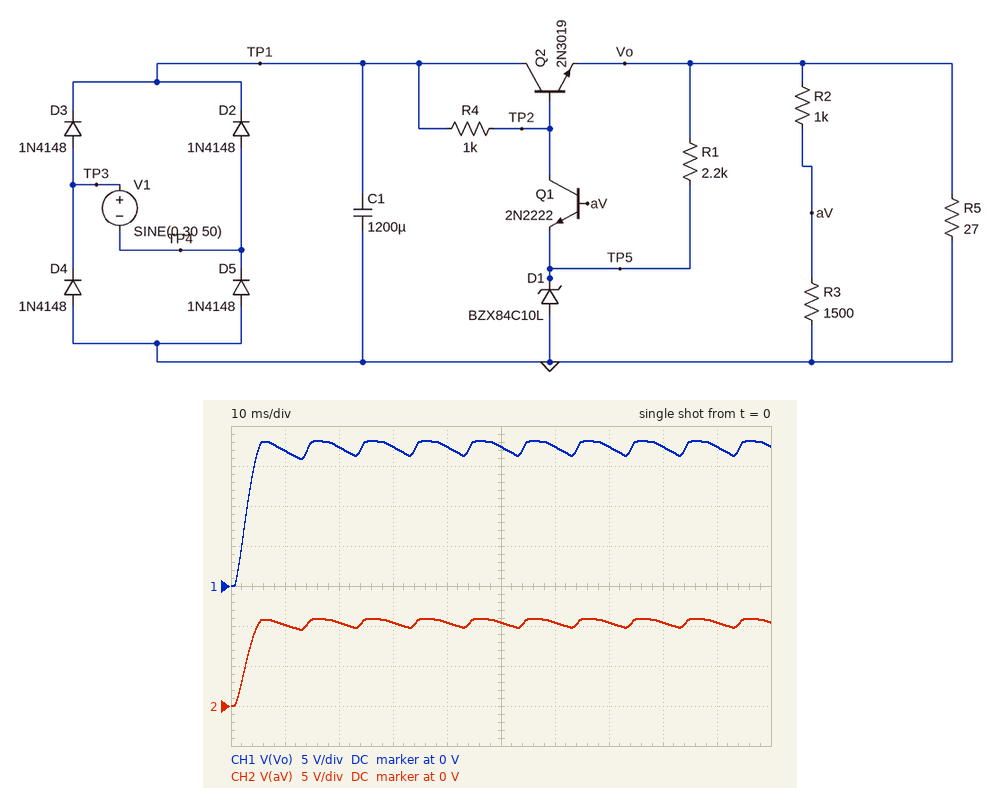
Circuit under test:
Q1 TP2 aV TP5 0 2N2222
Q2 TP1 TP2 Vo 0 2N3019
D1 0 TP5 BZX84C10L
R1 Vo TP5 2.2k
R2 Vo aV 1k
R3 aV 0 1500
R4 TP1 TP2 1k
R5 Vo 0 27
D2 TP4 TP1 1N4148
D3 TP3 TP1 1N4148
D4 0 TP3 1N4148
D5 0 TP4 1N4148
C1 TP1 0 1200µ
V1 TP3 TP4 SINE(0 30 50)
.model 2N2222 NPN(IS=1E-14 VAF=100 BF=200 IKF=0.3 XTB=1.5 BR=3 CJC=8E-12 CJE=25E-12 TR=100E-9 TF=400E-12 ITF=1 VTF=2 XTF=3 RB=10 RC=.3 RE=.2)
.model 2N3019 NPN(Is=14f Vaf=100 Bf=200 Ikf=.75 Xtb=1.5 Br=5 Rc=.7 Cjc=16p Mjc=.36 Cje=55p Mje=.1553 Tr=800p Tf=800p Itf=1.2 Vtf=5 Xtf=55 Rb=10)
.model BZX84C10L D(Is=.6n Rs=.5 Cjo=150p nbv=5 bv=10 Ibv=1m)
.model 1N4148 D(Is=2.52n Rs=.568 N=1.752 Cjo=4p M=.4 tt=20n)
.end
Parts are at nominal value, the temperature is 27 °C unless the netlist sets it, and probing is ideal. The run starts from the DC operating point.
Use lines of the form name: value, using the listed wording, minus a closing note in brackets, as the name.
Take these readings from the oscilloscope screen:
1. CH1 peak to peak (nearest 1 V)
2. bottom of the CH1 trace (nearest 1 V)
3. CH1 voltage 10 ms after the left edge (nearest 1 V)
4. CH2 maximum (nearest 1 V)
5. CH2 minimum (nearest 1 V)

CH1 peak to peak: 18 V
bottom of the CH1 trace: 0 V
CH1 voltage 10 ms after the left edge: 17 V
CH2 maximum: 11 V
CH2 minimum: 0 V
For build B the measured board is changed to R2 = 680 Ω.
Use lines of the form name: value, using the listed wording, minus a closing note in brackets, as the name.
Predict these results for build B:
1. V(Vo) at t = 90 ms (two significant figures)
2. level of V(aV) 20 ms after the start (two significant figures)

V(Vo) at t = 90 ms: 16 V
level of V(aV) 20 ms after the start: 11 V
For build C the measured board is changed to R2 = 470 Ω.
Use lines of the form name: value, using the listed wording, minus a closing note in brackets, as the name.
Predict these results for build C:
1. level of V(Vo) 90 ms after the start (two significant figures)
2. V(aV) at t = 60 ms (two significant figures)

level of V(Vo) 90 ms after the start: 14 V
V(aV) at t = 60 ms: 11 V
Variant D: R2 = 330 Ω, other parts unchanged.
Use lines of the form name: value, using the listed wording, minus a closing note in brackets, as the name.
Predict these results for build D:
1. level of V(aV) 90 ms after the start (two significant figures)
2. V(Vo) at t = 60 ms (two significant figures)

level of V(aV) 90 ms after the start: 11 V
V(Vo) at t = 60 ms: 13 V
